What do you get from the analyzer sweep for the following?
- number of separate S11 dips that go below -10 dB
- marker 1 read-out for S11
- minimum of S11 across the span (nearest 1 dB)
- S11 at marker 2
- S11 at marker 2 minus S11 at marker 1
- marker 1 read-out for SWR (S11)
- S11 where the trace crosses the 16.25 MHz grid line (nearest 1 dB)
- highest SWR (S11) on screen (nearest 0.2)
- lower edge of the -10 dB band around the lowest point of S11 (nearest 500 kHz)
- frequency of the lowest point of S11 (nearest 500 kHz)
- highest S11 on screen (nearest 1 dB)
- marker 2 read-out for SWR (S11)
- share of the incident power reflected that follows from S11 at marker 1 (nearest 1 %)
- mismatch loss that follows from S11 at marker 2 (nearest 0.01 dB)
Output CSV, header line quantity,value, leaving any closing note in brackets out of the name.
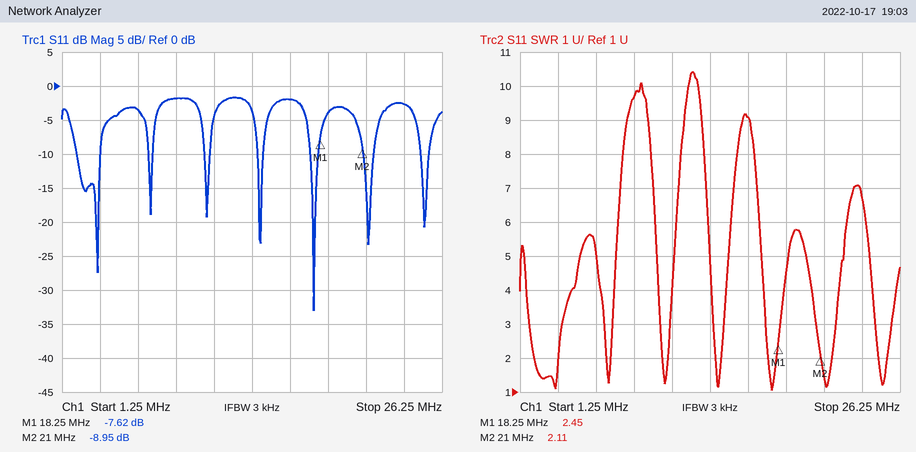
quantity,value
number of separate S11 dips that go below -10 dB,7
marker 1 read-out for S11,-7.62 dB
minimum of S11 across the span,-33 dB
S11 at marker 2,-8.95 dB
S11 at marker 2 minus S11 at marker 1,-1.33 dB
marker 1 read-out for SWR,2.45
S11 where the trace crosses the 16.25 MHz grid line,-2 dB
highest SWR (S11) on screen,10.4
lower edge of the -10 dB band around the lowest point of S11,17.5 MHz
frequency of the lowest point of S11,18.0 MHz
highest S11 on screen,-2 dB
marker 2 read-out for SWR,2.11
share of the incident power reflected that follows from S11 at marker 1,17 %
mismatch loss that follows from S11 at marker 2,0.59 dB
